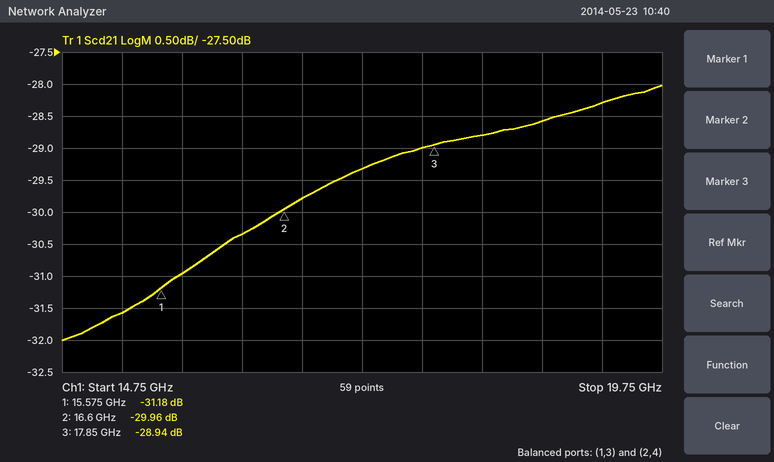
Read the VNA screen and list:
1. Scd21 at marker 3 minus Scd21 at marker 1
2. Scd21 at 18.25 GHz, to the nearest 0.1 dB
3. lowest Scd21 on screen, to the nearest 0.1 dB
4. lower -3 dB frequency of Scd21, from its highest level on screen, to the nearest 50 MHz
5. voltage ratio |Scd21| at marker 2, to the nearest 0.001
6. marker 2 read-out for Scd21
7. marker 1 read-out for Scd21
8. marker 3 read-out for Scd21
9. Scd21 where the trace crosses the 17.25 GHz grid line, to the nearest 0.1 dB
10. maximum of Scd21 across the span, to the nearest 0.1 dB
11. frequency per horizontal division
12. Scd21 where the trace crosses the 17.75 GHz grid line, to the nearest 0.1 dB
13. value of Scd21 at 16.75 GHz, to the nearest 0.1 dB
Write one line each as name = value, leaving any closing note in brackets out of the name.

Scd21 at marker 3 minus Scd21 at marker 1 = 2.24 dB
Scd21 at 18.25 GHz, to the nearest 0.1 dB = -28.8 dB
lowest Scd21 on screen, to the nearest 0.1 dB = -32.0 dB
lower -3 dB frequency of Scd21, from its highest level on screen, to the nearest 50 MHz = 15.70 GHz
voltage ratio |Scd21| at marker 2, to the nearest 0.001 = 0.032
marker 2 read-out for Scd21 = -29.96 dB
marker 1 read-out for Scd21 = -31.18 dB
marker 3 read-out for Scd21 = -28.94 dB
Scd21 where the trace crosses the 17.25 GHz grid line, to the nearest 0.1 dB = -29.3 dB
maximum of Scd21 across the span, to the nearest 0.1 dB = -28.0 dB
frequency per horizontal division = 500 MHz
Scd21 where the trace crosses the 17.75 GHz grid line, to the nearest 0.1 dB = -29.0 dB
value of Scd21 at 16.75 GHz, to the nearest 0.1 dB = -29.8 dB
